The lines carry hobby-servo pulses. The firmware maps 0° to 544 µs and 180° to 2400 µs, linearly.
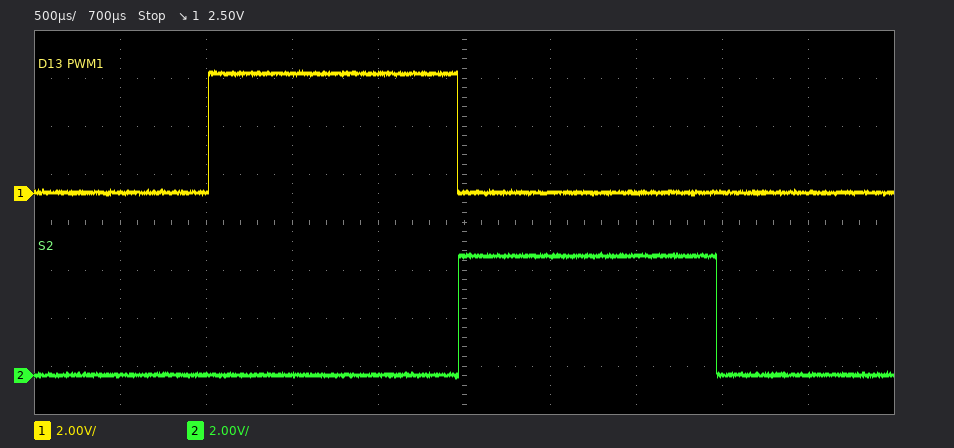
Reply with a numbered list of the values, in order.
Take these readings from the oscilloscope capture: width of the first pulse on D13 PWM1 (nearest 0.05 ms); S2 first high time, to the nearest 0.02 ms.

1. 1.45 ms
2. 1.50 ms
